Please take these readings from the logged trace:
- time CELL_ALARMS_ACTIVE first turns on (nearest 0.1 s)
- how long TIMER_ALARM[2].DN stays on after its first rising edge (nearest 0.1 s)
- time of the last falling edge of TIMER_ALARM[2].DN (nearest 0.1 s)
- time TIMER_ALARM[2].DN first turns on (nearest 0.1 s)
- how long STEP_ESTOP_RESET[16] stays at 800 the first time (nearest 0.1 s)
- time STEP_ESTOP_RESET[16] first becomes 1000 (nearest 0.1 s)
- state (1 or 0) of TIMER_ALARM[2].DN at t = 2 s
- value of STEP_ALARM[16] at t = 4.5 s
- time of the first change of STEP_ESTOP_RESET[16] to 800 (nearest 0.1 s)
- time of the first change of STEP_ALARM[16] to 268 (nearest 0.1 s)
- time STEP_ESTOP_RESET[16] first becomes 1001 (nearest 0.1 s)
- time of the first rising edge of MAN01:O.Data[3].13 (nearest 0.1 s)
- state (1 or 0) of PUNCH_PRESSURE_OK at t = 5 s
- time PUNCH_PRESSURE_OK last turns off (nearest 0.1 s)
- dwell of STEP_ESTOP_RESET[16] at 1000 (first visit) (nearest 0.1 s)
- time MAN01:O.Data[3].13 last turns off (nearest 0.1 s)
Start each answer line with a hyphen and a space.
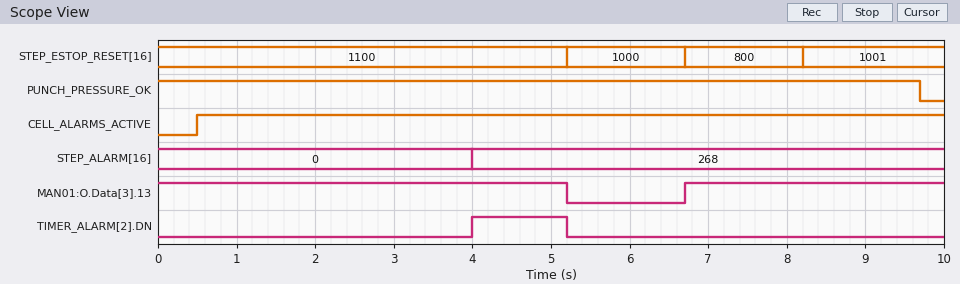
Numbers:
- 0.5 s
- 1.2 s
- 5.2 s
- 4.0 s
- 1.5 s
- 5.2 s
- 0
- 268
- 6.7 s
- 4.0 s
- 8.2 s
- 6.7 s
- 1
- 9.7 s
- 1.5 s
- 5.2 s
